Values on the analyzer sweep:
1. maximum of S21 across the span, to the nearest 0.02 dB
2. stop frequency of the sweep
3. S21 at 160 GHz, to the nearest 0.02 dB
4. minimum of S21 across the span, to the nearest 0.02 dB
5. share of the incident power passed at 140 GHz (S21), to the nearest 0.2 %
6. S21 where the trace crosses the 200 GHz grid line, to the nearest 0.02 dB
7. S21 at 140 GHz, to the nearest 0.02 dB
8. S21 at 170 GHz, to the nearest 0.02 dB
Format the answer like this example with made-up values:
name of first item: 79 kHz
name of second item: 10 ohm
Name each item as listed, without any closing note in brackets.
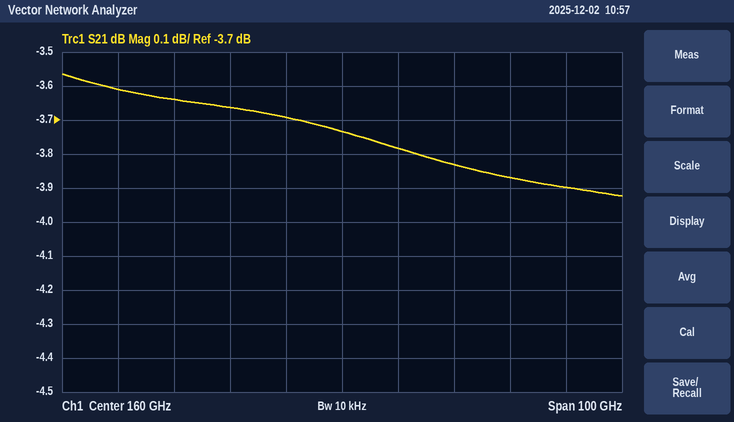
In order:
maximum of S21 across the span, to the nearest 0.02 dB: -3.56 dB
stop frequency of the sweep: 210 GHz
S21 at 160 GHz, to the nearest 0.02 dB: -3.74 dB
minimum of S21 across the span, to the nearest 0.02 dB: -3.92 dB
share of the incident power passed at 140 GHz (S21), to the nearest 0.2 %: 43.0 %
S21 where the trace crosses the 200 GHz grid line, to the nearest 0.02 dB: -3.90 dB
S21 at 140 GHz, to the nearest 0.02 dB: -3.66 dB
S21 at 170 GHz, to the nearest 0.02 dB: -3.78 dB
